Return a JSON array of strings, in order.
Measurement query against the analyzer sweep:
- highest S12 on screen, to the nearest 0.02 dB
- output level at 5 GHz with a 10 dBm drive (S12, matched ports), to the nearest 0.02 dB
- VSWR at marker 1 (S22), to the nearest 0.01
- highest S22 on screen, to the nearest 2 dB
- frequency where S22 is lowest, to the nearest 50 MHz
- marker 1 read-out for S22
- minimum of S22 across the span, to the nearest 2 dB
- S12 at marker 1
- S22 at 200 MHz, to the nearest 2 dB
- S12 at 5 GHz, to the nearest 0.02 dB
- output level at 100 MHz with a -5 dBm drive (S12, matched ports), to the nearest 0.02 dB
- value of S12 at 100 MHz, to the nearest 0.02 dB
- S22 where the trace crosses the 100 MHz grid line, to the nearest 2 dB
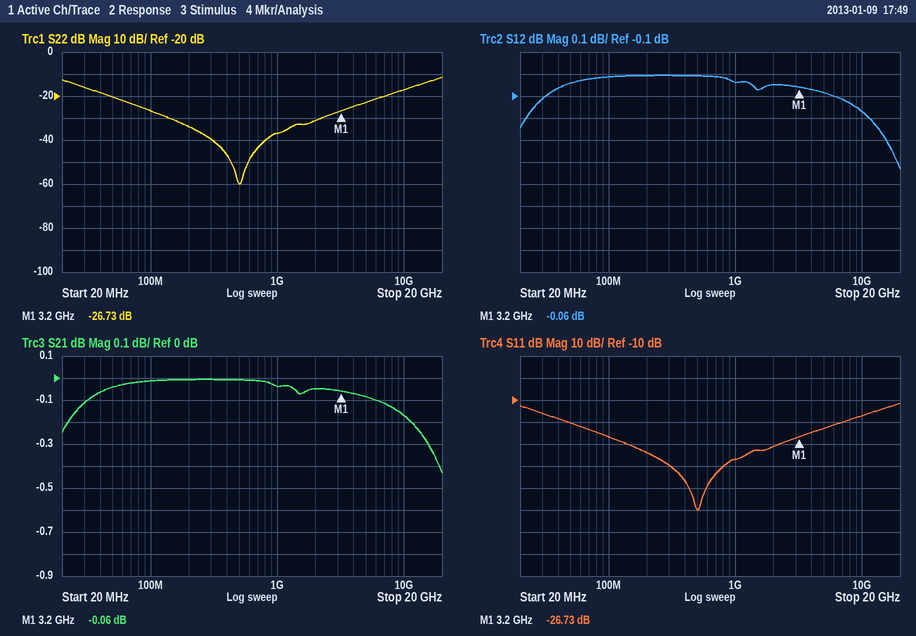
["0.00 dB", "9.92 dBm", "1.10", "-12 dB", "500 MHz", "-26.73 dB", "-60 dB", "-0.06 dB", "-34 dB", "-0.08 dB", "-5.02 dBm", "-0.02 dB", "-26 dB"]
